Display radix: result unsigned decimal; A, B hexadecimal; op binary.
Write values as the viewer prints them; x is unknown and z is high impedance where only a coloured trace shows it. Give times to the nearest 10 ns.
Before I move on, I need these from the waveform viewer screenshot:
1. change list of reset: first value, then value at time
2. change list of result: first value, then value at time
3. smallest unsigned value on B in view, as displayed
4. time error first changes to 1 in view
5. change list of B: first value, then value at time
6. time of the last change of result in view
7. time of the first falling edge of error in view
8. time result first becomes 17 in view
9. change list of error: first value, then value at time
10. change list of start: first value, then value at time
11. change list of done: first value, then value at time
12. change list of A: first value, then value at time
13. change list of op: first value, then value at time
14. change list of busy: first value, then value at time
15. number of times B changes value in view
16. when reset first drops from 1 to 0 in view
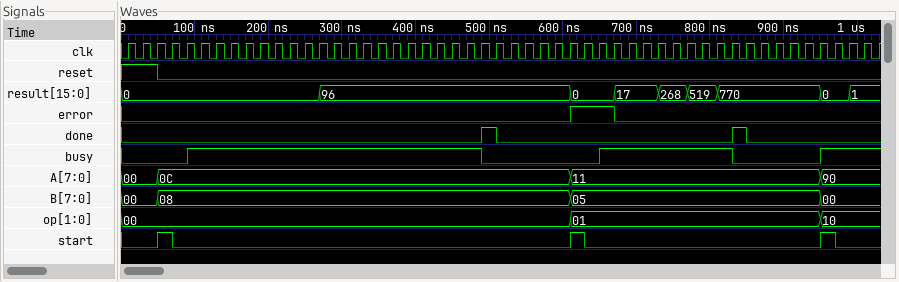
1, 0 at 50 ns
0, 96 at 270 ns, 0 at 610 ns, 17 at 670 ns, 268 at 730 ns, 519 at 770 ns, 770 at 810 ns, 0 at 950 ns, 1 at 990 ns
00
610 ns
00, 08 at 50 ns, 05 at 610 ns, 00 at 950 ns
990 ns
670 ns
670 ns
0, 1 at 610 ns, 0 at 670 ns
0, 1 at 50 ns, 0 at 70 ns, 1 at 610 ns, 0 at 630 ns, 1 at 950 ns, 0 at 970 ns
0, 1 at 490 ns, 0 at 510 ns, 1 at 830 ns, 0 at 850 ns
00, 0C at 50 ns, 11 at 610 ns, 90 at 950 ns
00, 01 at 610 ns, 10 at 950 ns
0, 1 at 90 ns, 0 at 490 ns, 1 at 650 ns, 0 at 830 ns, 1 at 950 ns
3
50 ns
